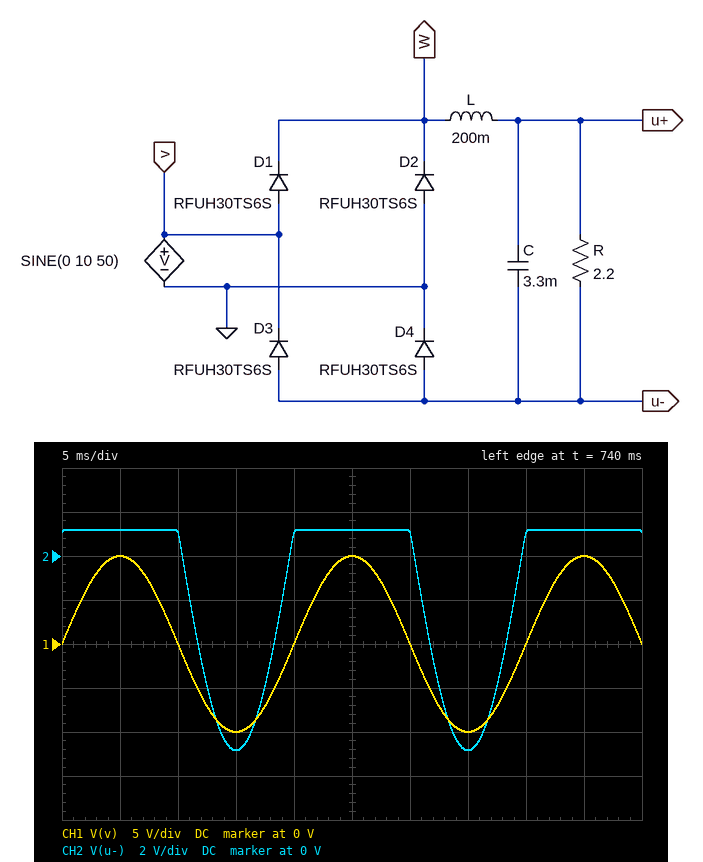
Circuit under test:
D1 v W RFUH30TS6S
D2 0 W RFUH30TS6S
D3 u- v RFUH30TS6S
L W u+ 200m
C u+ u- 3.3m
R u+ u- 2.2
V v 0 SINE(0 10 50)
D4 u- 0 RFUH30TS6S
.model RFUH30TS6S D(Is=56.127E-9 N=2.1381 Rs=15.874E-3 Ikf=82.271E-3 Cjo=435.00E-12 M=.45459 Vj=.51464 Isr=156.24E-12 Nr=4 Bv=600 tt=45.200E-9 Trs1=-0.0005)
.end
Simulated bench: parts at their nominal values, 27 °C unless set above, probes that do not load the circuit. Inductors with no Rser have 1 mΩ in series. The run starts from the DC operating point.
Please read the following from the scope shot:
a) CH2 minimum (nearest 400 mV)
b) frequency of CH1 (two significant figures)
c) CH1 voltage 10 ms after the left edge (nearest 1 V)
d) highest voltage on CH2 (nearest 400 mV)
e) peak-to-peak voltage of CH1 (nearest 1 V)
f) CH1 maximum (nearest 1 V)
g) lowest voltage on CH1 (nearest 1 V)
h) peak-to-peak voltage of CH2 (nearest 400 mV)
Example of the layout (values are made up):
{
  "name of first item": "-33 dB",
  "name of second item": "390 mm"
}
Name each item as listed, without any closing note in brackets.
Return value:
{
  "CH2 minimum": "-8.8 V",
  "frequency of CH1": "50 Hz",
  "CH1 voltage 10 ms after the left edge": "0 V",
  "highest voltage on CH2": "1.2 V",
  "peak-to-peak voltage of CH1": "20 V",
  "CH1 maximum": "10 V",
  "lowest voltage on CH1": "-10 V",
  "peak-to-peak voltage of CH2": "10.0 V"
}
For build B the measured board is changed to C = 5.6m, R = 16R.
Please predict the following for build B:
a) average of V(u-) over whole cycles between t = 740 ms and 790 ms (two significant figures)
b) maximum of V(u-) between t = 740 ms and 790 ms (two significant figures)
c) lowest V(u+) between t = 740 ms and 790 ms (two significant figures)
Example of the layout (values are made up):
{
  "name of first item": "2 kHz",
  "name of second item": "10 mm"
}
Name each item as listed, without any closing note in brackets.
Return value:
{
  "average of V(u-) over whole cycles between t = 740 ms and 790 ms": "-2.2 V",
  "maximum of V(u-) between t = 740 ms and 790 ms": "960 mV",
  "lowest V(u+) between t = 740 ms and 790 ms": "-4.6 V"
}
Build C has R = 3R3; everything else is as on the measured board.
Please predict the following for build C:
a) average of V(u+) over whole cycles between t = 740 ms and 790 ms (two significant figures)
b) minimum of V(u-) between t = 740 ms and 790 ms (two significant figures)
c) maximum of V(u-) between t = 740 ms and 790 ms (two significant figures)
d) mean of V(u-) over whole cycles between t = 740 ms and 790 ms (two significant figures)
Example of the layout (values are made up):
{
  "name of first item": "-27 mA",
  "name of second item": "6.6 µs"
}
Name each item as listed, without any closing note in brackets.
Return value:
{
  "average of V(u+) over whole cycles between t = 740 ms and 790 ms": "2.1 V",
  "minimum of V(u-) between t = 740 ms and 790 ms": "-8.9 V",
  "maximum of V(u-) between t = 740 ms and 790 ms": "1.1 V",
  "mean of V(u-) over whole cycles between t = 740 ms and 790 ms": "-2.1 V"
}
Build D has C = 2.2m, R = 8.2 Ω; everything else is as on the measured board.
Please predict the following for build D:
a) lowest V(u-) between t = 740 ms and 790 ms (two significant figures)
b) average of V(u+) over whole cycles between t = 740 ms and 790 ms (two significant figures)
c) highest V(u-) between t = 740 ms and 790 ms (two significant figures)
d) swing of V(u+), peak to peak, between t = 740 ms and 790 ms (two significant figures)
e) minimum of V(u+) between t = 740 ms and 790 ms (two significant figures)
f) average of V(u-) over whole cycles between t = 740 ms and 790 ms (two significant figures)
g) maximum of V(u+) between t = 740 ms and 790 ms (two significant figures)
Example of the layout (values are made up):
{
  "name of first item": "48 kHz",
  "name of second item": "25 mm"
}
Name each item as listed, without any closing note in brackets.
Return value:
{
  "lowest V(u-) between t = 740 ms and 790 ms": "-9.0 V",
  "average of V(u+) over whole cycles between t = 740 ms and 790 ms": "2.2 V",
  "highest V(u-) between t = 740 ms and 790 ms": "1.0 V",
  "swing of V(u+), peak to peak, between t = 740 ms and 790 ms": "10 V",
  "minimum of V(u+) between t = 740 ms and 790 ms": "-4.7 V",
  "average of V(u-) over whole cycles between t = 740 ms and 790 ms": "-2.2 V",
  "maximum of V(u+) between t = 740 ms and 790 ms": "5.4 V"
}
